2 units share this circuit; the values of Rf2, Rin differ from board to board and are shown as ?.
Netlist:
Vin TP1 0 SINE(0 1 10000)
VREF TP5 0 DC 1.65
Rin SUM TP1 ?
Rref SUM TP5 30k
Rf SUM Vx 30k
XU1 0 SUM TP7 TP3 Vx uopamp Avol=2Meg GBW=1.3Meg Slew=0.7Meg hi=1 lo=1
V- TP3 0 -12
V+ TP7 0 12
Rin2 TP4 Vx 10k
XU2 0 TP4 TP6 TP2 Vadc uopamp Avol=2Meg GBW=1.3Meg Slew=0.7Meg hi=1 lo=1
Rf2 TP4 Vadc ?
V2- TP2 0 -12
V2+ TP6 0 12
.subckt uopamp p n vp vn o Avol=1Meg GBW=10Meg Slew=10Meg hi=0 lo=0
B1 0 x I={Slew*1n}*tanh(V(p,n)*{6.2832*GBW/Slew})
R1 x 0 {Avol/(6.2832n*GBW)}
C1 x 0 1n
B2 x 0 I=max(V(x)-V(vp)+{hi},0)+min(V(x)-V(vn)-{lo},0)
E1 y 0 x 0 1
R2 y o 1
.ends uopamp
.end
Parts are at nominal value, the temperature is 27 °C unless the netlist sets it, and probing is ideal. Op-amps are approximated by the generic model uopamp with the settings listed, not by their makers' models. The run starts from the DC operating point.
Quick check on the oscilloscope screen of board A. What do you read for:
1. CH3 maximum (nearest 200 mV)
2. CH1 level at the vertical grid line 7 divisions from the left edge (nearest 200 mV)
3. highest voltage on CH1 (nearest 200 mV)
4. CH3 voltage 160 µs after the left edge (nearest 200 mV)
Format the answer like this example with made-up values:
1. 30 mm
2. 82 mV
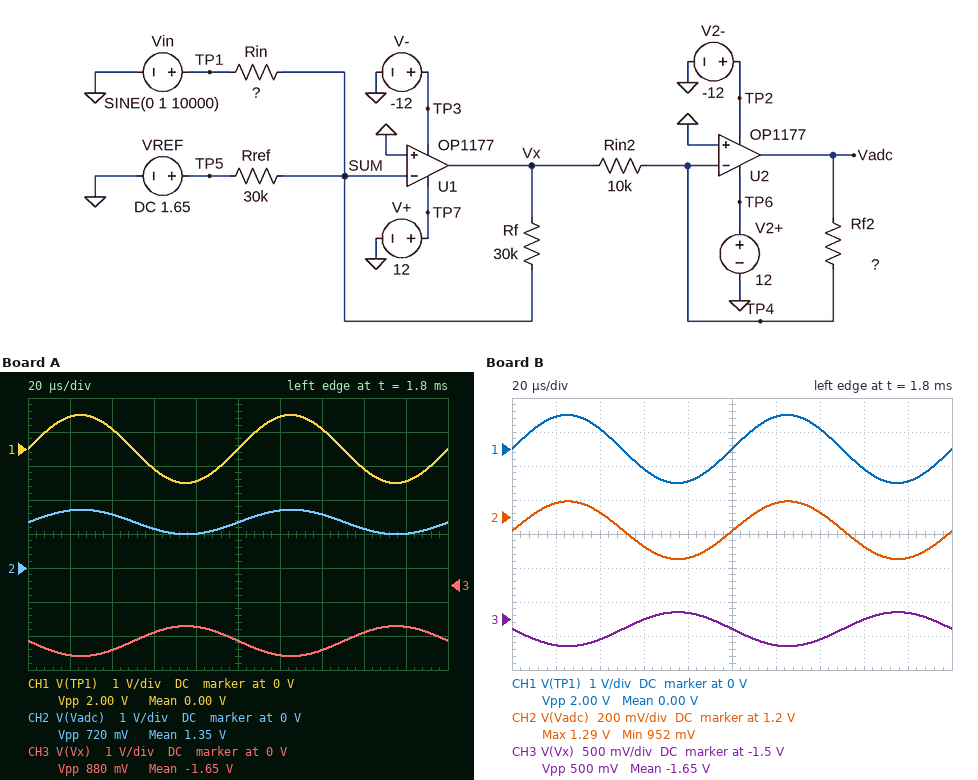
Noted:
1. -1.2 V
2. 600 mV
3. 1.0 V
4. -1.4 V
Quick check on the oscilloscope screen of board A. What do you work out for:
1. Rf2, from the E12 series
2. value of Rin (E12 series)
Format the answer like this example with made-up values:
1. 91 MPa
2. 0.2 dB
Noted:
1. 8.2 kΩ
2. 68 kΩ
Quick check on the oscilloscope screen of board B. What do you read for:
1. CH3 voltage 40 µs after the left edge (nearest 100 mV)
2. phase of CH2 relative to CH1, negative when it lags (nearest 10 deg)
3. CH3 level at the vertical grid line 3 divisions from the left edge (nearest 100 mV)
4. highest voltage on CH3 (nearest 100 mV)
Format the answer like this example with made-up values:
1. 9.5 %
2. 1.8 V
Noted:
1. -1.8 V
2. 0 deg
3. -1.5 V
4. -1.4 V
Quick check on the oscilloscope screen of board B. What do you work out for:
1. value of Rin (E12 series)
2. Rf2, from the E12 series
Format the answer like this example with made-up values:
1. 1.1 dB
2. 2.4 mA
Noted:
1. 120 kΩ
2. 6.8 kΩ
